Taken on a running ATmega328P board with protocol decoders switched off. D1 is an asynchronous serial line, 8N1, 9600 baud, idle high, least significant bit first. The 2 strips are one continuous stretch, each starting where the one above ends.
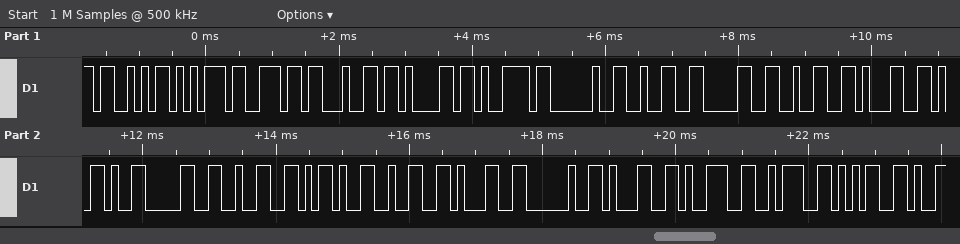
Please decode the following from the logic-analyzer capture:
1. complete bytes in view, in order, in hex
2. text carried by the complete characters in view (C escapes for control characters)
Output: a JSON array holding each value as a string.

["53 75 6E 64 61 79 20 32 30 32 31 2D 30 32 2D 32 31 20 31 39 3A 35", "\"Sunday 2021-02-21 19:5\""]
